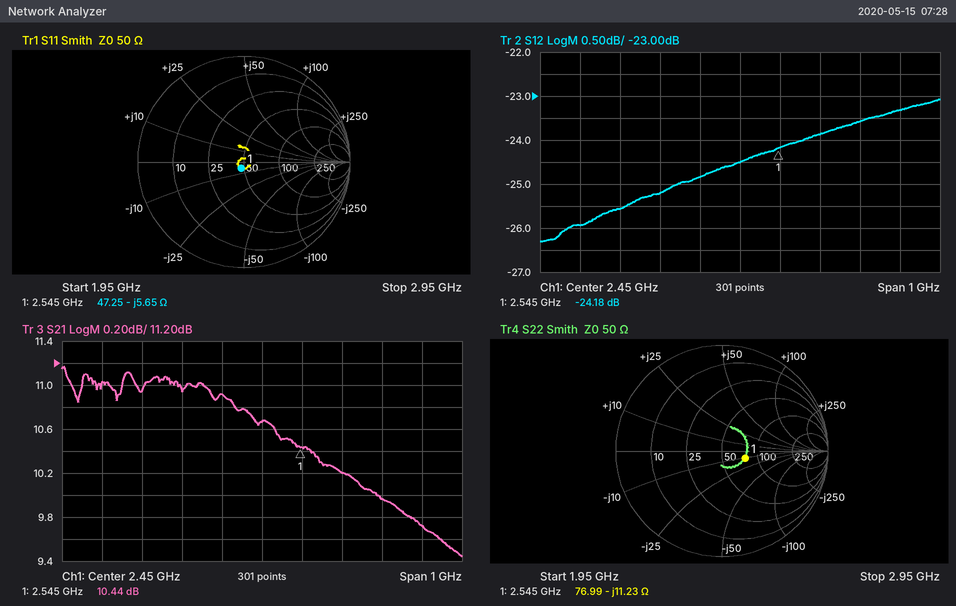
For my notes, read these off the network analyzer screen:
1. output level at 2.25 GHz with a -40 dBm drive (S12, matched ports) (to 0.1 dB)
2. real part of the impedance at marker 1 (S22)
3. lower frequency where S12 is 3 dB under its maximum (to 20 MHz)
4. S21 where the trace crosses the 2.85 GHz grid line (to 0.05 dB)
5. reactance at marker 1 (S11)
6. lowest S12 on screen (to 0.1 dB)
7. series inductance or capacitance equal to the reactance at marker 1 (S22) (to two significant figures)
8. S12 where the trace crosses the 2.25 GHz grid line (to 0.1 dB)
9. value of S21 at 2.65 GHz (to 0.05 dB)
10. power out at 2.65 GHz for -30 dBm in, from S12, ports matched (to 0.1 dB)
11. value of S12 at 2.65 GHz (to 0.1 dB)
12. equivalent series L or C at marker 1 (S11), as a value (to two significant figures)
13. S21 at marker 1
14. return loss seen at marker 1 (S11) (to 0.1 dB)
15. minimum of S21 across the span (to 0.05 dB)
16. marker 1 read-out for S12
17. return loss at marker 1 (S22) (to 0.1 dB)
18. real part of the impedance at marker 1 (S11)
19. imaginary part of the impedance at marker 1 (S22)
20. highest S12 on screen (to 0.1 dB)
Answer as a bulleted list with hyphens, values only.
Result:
- -65.2 dBm
- 76.99 Ω
- 2.00 GHz
- 9.70 dB
- -5.65 Ω
- -26.3 dB
- 5.6 pF
- -25.2 dB
- 10.20 dB
- -53.9 dBm
- -23.9 dB
- 11 pF
- 10.44 dB
- 23.8 dB
- 9.45 dB
- -24.18 dB
- 12.8 dB
- 47.25 Ω
- -11.23 Ω
- -23.1 dB
